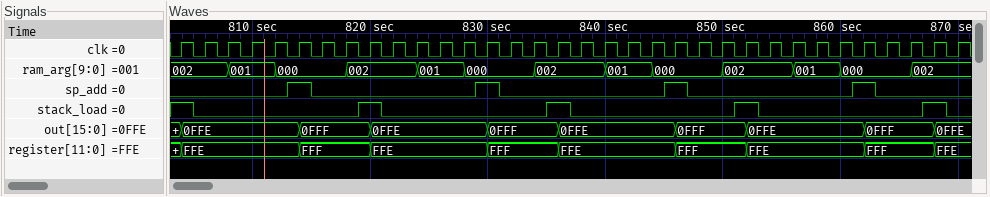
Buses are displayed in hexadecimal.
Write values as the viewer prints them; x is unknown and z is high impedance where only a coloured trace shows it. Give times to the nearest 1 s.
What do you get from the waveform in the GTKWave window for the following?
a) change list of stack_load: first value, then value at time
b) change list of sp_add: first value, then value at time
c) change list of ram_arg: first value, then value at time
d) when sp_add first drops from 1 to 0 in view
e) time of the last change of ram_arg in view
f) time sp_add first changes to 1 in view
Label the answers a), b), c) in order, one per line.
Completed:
a) 1, 0 at 805 s, 1 at 819 s, 0 at 821 s, 1 at 835 s, 0 at 837 s, 1 at 851 s, 0 at 853 s, 1 at 867 s, 0 at 869 s
b) 0, 1 at 813 s, 0 at 815 s, 1 at 829 s, 0 at 831 s, 1 at 845 s, 0 at 847 s, 1 at 861 s, 0 at 863 s
c) 002, 001 at 808 s, 000 at 812 s, 002 at 818 s, 001 at 824 s, 000 at 828 s, 002 at 834 s, 001 at 840 s, 000 at 844 s, 002 at 850 s, 001 at 856 s, 000 at 860 s, 002 at 866 s
d) 815 s
e) 866 s
f) 813 s
